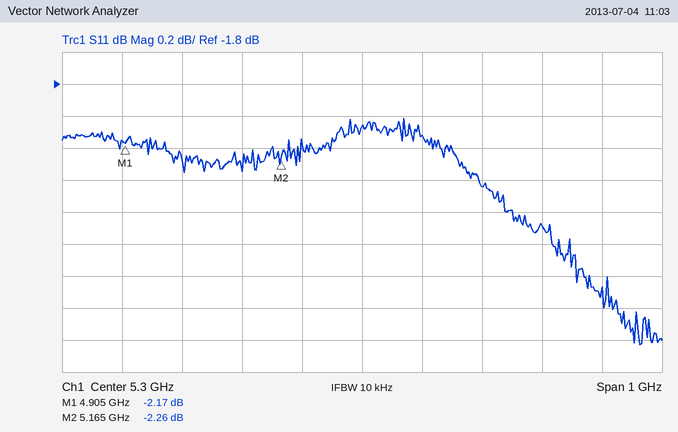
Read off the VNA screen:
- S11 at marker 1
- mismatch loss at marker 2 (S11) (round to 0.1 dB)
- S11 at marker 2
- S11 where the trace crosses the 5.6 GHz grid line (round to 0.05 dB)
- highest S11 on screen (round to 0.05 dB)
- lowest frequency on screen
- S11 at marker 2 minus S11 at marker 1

-2.17 dB
3.9 dB
-2.26 dB
-2.70 dB
-2.00 dB
4.8 GHz
-0.09 dB
